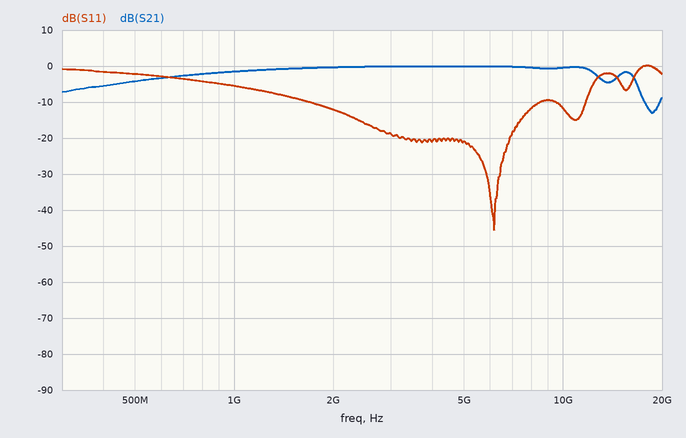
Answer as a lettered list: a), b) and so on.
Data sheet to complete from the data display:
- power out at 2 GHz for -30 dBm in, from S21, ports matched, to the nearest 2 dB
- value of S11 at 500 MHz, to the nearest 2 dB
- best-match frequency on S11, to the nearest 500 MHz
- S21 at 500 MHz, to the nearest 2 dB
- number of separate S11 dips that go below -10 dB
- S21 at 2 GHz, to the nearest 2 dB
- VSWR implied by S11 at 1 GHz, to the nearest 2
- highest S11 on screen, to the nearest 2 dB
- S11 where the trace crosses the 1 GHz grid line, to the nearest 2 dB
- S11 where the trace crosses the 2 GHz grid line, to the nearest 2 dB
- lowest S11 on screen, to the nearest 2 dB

a) -30 dBm
b) -2 dB
c) 6.0 GHz
d) -4 dB
e) 2
f) 0 dB
g) 4
h) 0 dB
i) -6 dB
j) -12 dB
k) -46 dB
